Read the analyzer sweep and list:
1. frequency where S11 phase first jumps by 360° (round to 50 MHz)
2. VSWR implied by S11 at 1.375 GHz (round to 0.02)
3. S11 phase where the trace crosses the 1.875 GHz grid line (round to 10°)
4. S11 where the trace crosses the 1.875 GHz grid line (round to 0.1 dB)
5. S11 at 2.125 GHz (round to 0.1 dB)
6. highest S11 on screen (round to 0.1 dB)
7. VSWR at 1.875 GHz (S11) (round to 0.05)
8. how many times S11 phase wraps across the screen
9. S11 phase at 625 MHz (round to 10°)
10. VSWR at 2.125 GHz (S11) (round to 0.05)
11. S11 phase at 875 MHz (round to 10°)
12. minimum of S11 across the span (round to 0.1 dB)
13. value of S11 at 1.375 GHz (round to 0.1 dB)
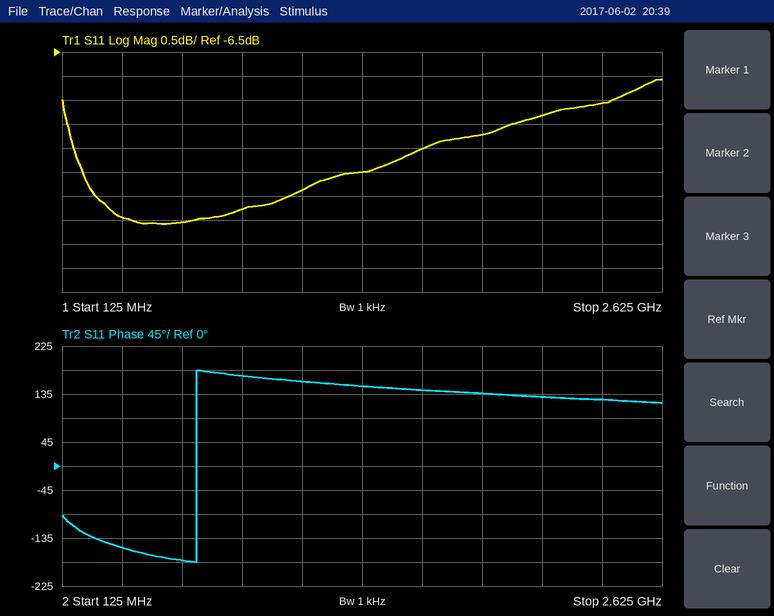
700 MHz
2.10
140°
-8.2 dB
-7.8 dB
-7.1 dB
2.25
1
-180°
2.35
170°
-10.1 dB
-9.0 dB
